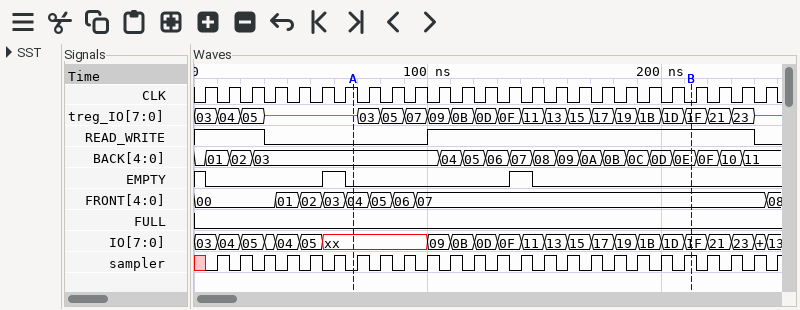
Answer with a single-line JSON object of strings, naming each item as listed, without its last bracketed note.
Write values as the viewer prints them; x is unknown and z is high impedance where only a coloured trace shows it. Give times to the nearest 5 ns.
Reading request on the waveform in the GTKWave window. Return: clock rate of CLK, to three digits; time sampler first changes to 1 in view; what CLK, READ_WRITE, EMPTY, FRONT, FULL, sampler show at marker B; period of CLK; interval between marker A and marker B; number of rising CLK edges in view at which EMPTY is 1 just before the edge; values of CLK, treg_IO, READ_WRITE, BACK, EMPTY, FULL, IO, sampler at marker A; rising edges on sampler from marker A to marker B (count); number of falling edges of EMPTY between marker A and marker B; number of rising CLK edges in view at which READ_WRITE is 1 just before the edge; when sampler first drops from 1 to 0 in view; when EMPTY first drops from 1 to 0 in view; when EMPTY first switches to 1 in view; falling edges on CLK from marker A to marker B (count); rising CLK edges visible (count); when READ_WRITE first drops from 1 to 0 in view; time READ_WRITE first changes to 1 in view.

{"clock rate of CLK, to three digits": "100 MHz", "time sampler first changes to 1 in view": "10 ns", "what CLK, READ_WRITE, EMPTY, FRONT, FULL, sampler show at marker B": "CLK=0, READ_WRITE=1, EMPTY=0, FRONT=07, FULL=0, sampler=1", "period of CLK": "10 ns", "interval between marker A and marker B": "145 ns", "number of rising CLK edges in view at which EMPTY is 1 just before the edge": "3", "values of CLK, treg_IO, READ_WRITE, BACK, EMPTY, FULL, IO, sampler at marker A": "CLK=1, treg_IO=z, READ_WRITE=0, BACK=03, EMPTY=0, FULL=0, IO=xx, sampler=0", "rising edges on sampler from marker A to marker B": "15", "number of falling edges of EMPTY between marker A and marker B": "1", "number of rising CLK edges in view at which READ_WRITE is 1 just before the edge": "17", "when sampler first drops from 1 to 0 in view": "15 ns", "when EMPTY first drops from 1 to 0 in view": "5 ns", "when EMPTY first switches to 1 in view": "55 ns", "falling edges on CLK from marker A to marker B": "15", "rising CLK edges visible": "25", "when READ_WRITE first drops from 1 to 0 in view": "30 ns", "time READ_WRITE first changes to 1 in view": "100 ns"}
